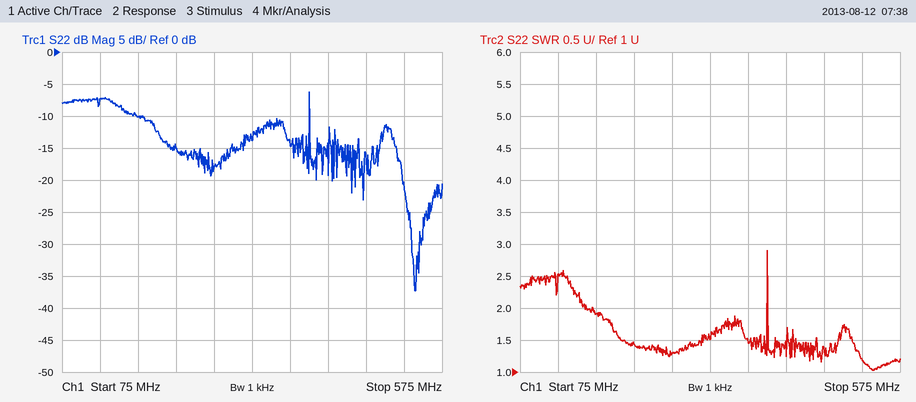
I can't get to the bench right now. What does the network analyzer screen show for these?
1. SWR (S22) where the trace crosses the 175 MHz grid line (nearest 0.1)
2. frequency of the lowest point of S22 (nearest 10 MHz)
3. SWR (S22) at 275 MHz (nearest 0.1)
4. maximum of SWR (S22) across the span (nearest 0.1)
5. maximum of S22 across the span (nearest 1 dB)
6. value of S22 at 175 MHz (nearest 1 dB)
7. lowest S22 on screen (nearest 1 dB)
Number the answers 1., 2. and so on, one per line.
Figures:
1. 1.9
2. 540 MHz
3. 1.3
4. 2.9
5. -6 dB
6. -10 dB
7. -37 dB
